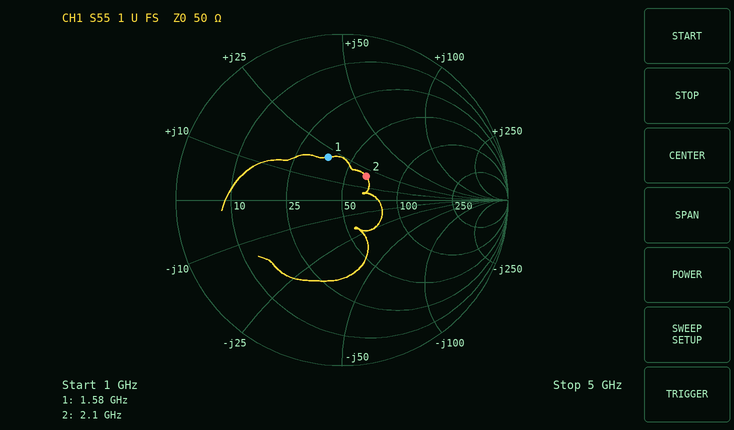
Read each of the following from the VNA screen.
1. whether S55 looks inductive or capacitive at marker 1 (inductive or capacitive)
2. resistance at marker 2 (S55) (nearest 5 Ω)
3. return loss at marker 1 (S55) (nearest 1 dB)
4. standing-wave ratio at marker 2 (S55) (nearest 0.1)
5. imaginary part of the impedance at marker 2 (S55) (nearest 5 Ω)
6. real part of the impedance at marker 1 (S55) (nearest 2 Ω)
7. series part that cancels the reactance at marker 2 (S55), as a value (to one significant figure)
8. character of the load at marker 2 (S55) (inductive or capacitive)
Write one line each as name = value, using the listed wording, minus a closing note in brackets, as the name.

whether S55 looks inductive or capacitive at marker 1 = inductive
resistance at marker 2 (S55) = 65 Ω
return loss at marker 1 (S55) = 11 dB
standing-wave ratio at marker 2 (S55) = 1.5
imaginary part of the impedance at marker 2 (S55) = +20 Ω
real part of the impedance at marker 1 (S55) = 38 Ω
series part that cancels the reactance at marker 2 (S55), as a value = 4 pF
character of the load at marker 2 (S55) = inductive
